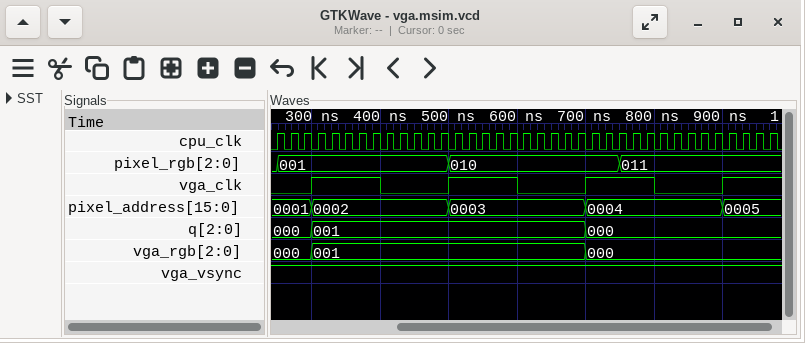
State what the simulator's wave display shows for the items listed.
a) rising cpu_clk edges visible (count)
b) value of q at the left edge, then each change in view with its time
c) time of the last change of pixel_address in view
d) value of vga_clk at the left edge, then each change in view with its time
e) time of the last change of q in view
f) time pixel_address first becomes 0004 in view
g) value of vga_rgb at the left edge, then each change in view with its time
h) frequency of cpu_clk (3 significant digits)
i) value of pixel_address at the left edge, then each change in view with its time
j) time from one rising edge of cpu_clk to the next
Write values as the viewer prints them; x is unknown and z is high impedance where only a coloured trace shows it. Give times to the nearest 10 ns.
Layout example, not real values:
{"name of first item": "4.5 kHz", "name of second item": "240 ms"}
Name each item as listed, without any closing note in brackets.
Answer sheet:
{"rising cpu_clk edges visible": "37", "value of q at the left edge, then each change in view with its time": "000, 001 at 300 ns, 000 at 700 ns", "time of the last change of pixel_address in view": "900 ns", "value of vga_clk at the left edge, then each change in view with its time": "0, 1 at 300 ns, 0 at 400 ns, 1 at 500 ns, 0 at 600 ns, 1 at 700 ns, 0 at 800 ns, 1 at 900 ns", "time of the last change of q in view": "700 ns", "time pixel_address first becomes 0004 in view": "700 ns", "value of vga_rgb at the left edge, then each change in view with its time": "000, 001 at 300 ns, 000 at 700 ns", "frequency of cpu_clk": "50.0 MHz", "value of pixel_address at the left edge, then each change in view with its time": "0001, 0002 at 300 ns, 0003 at 500 ns, 0004 at 700 ns, 0005 at 900 ns", "time from one rising edge of cpu_clk to the next": "20 ns"}
